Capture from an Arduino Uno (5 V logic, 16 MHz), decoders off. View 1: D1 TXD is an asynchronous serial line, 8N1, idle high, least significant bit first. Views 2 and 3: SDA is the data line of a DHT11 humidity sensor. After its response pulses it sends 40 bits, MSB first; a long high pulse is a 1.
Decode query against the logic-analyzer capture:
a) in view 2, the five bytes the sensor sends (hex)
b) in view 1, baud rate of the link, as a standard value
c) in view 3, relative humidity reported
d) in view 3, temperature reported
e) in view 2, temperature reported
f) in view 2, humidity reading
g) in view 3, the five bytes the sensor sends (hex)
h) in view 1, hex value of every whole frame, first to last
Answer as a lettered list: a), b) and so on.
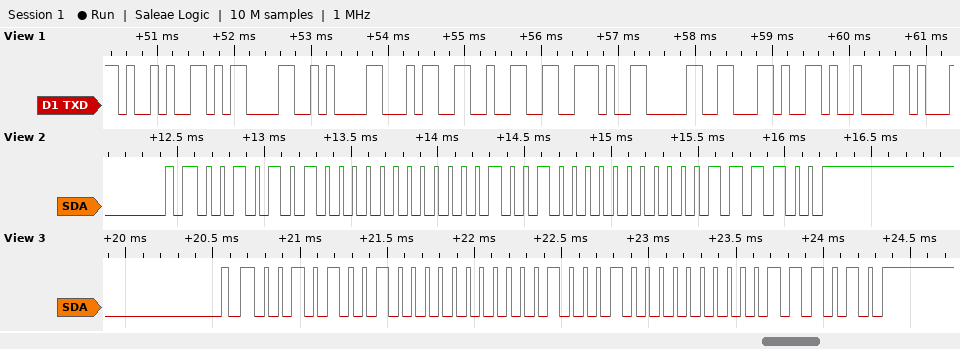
a) 2A 00 12 00 3C
b) 9600 baud
c) 41 %
d) 17.0 °C
e) 18.0 °C
f) 42 %
g) 29 00 11 00 3A
h) 0x29 0x0D 0x0A 0x34 0x32 0x2E 0x30 0x2C 0x09
